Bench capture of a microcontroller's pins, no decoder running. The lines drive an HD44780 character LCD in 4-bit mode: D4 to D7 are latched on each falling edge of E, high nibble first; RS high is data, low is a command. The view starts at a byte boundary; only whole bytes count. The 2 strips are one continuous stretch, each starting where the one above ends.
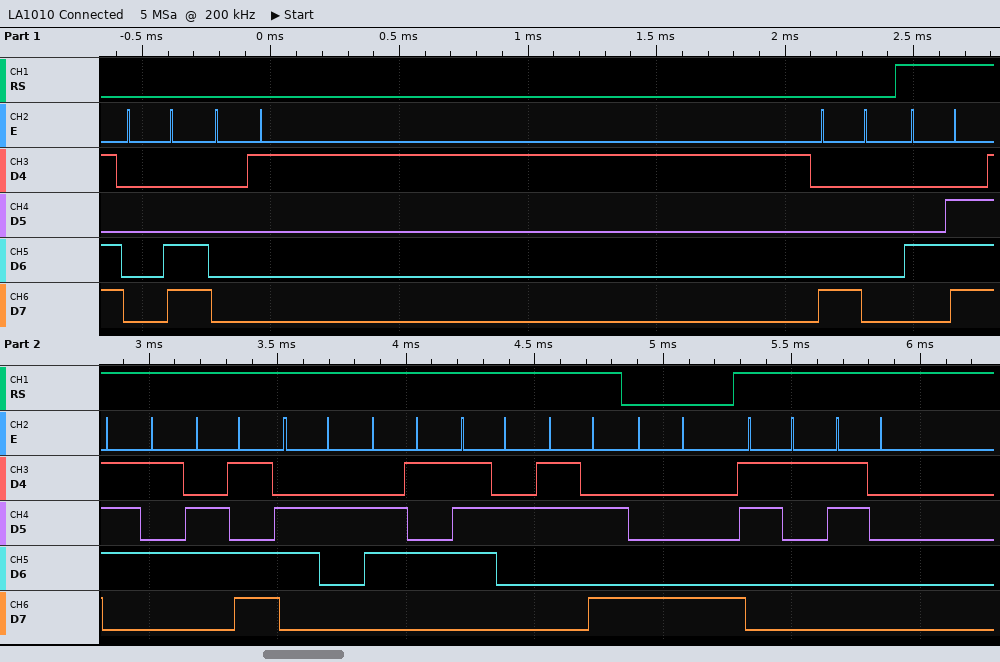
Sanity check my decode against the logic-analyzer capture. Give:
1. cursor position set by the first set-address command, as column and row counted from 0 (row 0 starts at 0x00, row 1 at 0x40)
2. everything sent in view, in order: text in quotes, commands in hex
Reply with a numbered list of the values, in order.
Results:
1. column 0, row 0
2. 0x0C 0x01 0x80 "Number:" 0x88 "10"
